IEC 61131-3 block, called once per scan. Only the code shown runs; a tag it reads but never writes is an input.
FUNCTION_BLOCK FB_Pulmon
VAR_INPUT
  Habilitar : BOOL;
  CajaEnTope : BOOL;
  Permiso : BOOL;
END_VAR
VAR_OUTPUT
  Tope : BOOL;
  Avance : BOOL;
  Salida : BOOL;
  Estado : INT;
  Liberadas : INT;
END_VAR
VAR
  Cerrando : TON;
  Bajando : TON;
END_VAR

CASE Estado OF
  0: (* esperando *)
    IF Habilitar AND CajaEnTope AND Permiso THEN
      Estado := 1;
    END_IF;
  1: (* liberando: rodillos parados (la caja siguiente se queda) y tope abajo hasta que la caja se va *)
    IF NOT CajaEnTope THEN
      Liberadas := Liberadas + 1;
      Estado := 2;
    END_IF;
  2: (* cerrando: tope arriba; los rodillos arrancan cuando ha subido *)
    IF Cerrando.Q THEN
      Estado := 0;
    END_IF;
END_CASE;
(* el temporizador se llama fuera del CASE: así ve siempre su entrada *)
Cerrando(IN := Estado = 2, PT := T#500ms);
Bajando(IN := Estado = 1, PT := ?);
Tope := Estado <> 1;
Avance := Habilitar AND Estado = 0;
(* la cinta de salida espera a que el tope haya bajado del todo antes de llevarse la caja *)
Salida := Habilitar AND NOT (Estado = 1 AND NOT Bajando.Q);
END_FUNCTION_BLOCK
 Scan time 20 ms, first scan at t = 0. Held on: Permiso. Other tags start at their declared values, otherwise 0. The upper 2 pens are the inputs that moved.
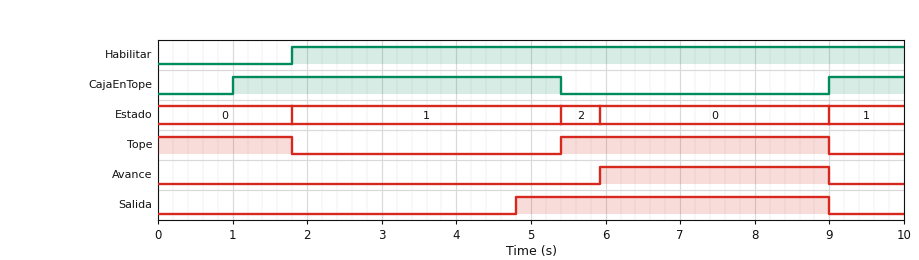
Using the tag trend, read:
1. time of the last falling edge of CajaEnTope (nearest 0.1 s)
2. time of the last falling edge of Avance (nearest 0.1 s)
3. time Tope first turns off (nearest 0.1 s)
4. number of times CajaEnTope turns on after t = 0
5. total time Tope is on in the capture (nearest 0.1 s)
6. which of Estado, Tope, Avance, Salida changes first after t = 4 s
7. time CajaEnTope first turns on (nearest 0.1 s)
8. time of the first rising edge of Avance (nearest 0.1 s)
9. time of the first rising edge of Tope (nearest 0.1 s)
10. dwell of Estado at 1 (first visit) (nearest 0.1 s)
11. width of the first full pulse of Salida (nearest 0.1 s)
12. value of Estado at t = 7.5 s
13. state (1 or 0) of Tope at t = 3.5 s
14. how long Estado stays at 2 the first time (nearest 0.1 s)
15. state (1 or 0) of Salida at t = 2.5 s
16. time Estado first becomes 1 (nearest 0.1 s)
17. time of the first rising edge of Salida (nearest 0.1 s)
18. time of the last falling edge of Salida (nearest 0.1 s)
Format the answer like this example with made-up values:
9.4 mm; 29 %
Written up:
5.4 s; 9.0 s; 1.8 s; 2; 5.4 s; Salida; 1.0 s; 5.9 s; 5.4 s; 3.6 s; 4.2 s; 0; 0; 0.5 s; 0; 1.8 s; 4.8 s; 9.0 s
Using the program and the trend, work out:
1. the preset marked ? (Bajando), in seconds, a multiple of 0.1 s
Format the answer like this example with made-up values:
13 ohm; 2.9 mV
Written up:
3.0 s
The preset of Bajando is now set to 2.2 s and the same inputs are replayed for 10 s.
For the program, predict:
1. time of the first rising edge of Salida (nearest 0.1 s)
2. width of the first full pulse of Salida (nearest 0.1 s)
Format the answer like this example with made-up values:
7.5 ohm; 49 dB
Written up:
4.0 s; 5.0 s
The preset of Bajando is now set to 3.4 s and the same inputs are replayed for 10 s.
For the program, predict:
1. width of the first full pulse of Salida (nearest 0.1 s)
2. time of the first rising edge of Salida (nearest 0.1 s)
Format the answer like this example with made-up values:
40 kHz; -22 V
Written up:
3.8 s; 5.2 s
